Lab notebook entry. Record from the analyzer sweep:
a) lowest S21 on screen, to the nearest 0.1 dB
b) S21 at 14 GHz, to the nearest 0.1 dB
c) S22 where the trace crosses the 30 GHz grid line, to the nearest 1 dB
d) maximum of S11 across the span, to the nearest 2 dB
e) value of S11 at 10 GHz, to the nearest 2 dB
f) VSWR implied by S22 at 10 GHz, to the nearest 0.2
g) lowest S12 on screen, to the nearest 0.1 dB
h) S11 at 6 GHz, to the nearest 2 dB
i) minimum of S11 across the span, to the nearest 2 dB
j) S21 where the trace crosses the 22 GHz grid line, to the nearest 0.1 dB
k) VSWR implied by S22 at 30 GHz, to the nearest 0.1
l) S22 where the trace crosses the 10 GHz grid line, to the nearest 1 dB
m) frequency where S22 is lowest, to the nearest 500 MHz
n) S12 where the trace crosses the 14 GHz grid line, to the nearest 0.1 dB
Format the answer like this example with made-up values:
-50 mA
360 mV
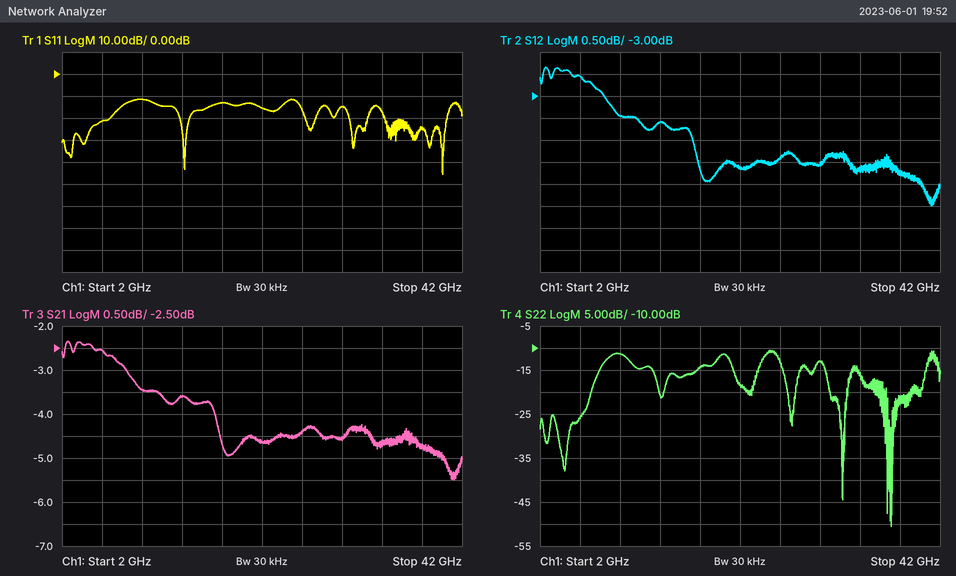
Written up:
-5.5 dB
-3.6 dB
-13 dB
-12 dB
-12 dB
1.8
-5.5 dB
-22 dB
-46 dB
-4.6 dB
1.6
-11 dB
37.0 GHz
-3.6 dB
